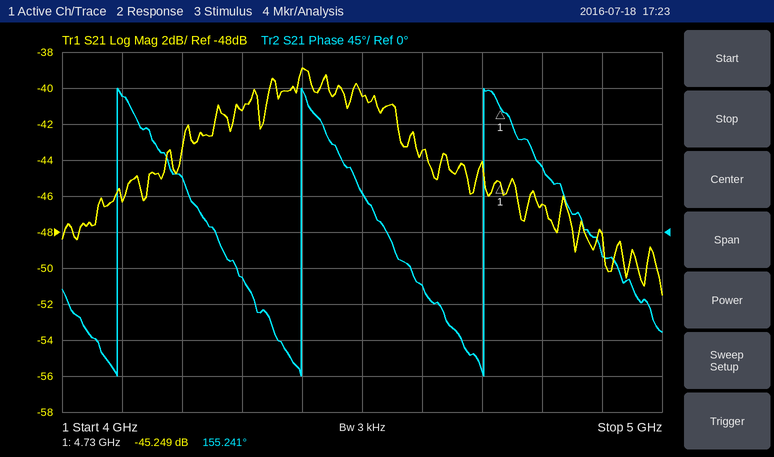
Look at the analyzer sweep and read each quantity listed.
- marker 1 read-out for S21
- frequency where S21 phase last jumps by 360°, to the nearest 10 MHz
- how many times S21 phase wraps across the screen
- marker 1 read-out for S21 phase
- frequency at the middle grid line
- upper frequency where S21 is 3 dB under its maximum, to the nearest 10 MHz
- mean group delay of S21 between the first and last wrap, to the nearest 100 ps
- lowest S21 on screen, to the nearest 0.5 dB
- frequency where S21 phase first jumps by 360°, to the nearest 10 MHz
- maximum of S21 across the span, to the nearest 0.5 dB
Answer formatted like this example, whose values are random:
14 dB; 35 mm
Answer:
-45.249 dB; 4.70 GHz; 3; 155.241°; 4.5 GHz; 4.56 GHz; 3.3 ns; -51.5 dB; 4.09 GHz; -39.0 dB
